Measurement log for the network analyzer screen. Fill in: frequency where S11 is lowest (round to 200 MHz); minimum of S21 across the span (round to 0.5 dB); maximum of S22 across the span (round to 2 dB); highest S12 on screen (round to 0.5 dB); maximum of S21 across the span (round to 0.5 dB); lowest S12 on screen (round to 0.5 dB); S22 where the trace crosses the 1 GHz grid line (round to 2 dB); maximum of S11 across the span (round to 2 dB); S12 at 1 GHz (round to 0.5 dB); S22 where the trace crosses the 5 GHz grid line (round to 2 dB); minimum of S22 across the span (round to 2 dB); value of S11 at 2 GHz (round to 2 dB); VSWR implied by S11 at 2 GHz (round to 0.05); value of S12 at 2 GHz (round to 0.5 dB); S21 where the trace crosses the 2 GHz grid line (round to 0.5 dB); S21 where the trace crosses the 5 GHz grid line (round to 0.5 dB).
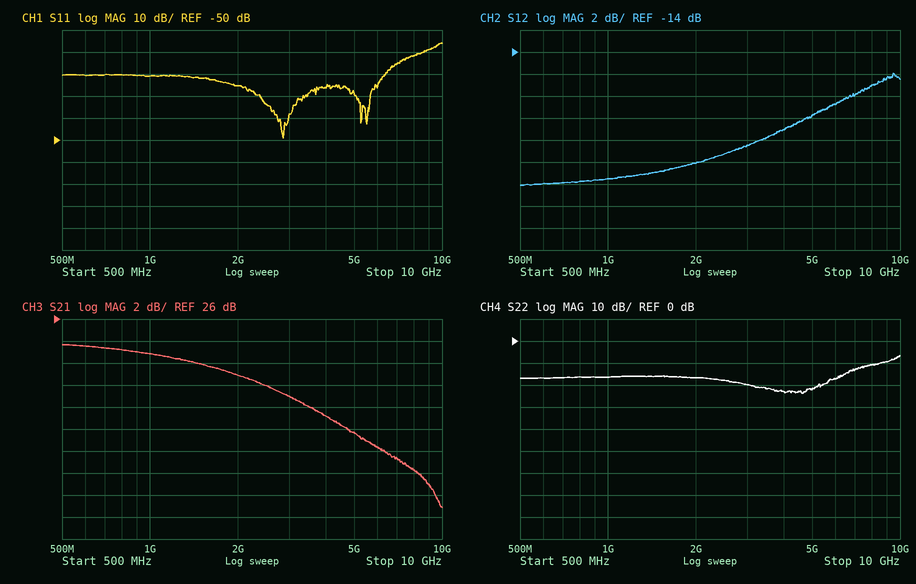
2.8 GHz
9.0 dB
-6 dB
-16.0 dB
23.5 dB
-26.0 dB
-16 dB
-6 dB
-25.5 dB
-22 dB
-24 dB
-26 dB
1.10
-24.0 dB
21.0 dB
15.5 dB
